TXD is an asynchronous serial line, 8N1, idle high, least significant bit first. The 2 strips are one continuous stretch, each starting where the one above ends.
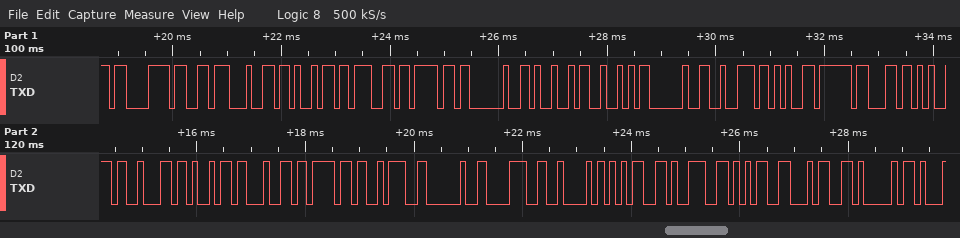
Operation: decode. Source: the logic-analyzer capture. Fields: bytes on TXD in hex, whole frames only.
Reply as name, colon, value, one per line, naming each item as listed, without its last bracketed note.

bytes on TXD in hex, whole frames only: 0xC3 0xB3 0x64 0x69 0x67 0x6F 0x20 0x49 0x52 0x20 0x72 0x65 0x63 0x65 0x62 0x69 0x64 0x6F 0x3A 0x20 0x38 0x42 0x35 0x39 0x35 0x34 0x41
